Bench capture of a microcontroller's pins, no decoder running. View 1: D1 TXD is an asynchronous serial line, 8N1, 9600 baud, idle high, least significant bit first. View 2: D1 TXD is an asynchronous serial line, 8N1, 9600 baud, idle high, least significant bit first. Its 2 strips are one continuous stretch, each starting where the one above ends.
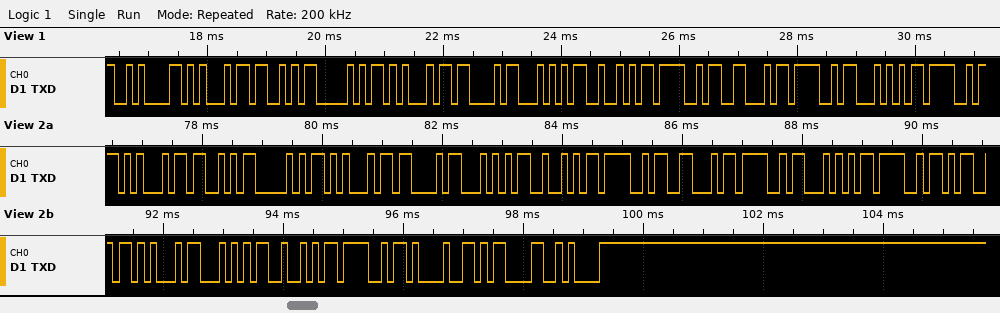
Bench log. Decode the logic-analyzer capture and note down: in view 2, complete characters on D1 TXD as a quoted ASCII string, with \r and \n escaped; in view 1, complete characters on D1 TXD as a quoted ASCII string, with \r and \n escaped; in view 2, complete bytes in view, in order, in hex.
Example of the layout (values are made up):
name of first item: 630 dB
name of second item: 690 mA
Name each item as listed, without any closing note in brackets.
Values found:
in view 2, complete characters on D1 TXD as a quoted ASCII string, with \r and \n escaped: "ESPECTROFOTOMETRO!\r\n"
in view 1, complete characters on D1 TXD as a quoted ASCII string, with \r and \n escaped: "\nESPECTROFOTO"
in view 2, complete bytes in view, in order, in hex: 45 53 50 45 43 54 52 4F 46 4F 54 4F 4D 45 54 52 4F 21 0D 0A
